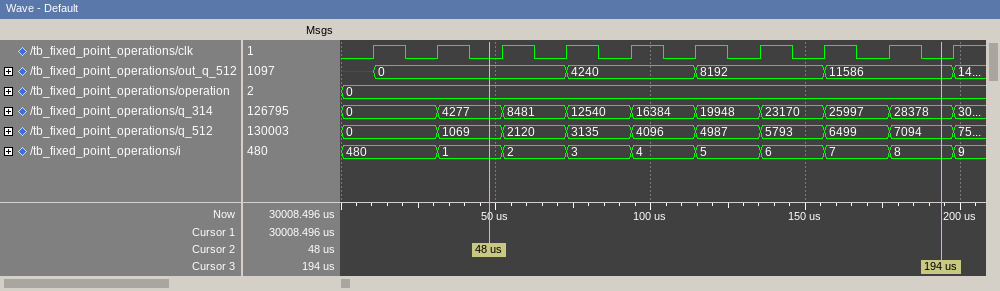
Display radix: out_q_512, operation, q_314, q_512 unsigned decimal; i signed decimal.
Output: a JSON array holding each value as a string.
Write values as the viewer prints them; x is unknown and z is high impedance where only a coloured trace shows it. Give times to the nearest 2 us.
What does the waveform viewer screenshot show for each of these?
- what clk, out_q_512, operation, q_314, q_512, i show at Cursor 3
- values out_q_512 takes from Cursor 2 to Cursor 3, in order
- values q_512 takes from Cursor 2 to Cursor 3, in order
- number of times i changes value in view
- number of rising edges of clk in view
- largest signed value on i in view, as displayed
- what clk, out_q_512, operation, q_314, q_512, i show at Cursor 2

["clk=0, out_q_512=11586, operation=0, q_314=28378, q_512=7094, i=8", "0, 4240, 8192, 11586", "1069, 2120, 3135, 4096, 4987, 5793, 6499, 7094", "9", "10", "480", "clk=0, out_q_512=0, operation=0, q_314=4277, q_512=1069, i=1"]
